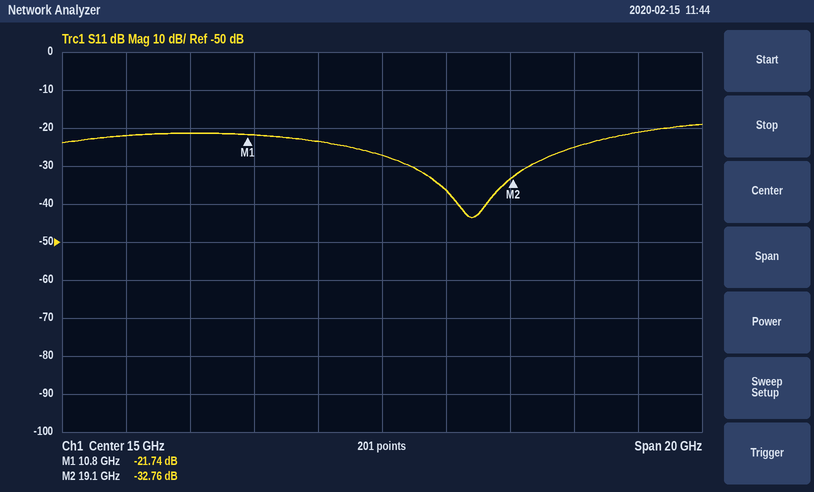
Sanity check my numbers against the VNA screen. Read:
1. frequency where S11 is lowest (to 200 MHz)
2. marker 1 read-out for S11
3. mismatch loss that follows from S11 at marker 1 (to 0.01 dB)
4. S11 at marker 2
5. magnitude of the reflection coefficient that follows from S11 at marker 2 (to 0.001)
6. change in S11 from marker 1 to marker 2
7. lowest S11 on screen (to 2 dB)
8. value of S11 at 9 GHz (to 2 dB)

17.8 GHz
-21.74 dB
0.03 dB
-32.76 dB
0.023
-11.02 dB
-44 dB
-22 dB
